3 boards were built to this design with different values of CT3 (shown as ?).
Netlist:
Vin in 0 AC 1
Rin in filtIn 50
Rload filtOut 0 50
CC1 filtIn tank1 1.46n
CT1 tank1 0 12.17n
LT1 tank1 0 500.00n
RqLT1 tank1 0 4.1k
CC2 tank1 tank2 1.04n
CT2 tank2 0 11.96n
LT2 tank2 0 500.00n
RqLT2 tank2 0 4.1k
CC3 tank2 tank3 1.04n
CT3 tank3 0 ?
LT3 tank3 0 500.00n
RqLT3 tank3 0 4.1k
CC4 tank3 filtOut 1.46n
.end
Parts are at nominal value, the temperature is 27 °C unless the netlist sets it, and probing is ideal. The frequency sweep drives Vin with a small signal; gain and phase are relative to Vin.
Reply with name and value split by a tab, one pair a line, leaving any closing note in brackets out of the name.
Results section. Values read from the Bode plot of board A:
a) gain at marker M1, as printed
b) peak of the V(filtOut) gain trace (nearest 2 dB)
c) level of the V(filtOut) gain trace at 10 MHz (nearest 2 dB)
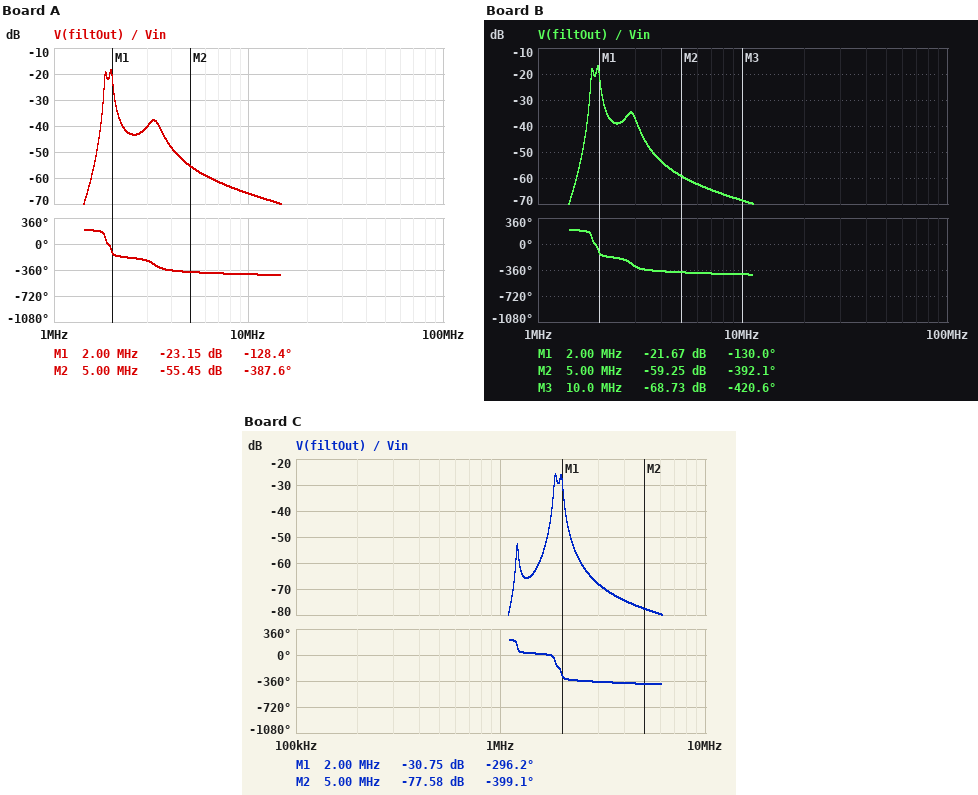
gain at marker M1, as printed	-23.15 dB
peak of the V(filtOut) gain trace	-18 dB
level of the V(filtOut) gain trace at 10 MHz	-66 dB
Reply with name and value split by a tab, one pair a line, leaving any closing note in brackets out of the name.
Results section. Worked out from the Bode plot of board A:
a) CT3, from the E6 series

CT3, from the E6 series	3.3 nF
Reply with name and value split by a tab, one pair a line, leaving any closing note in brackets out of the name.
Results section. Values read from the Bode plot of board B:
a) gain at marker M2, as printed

gain at marker M2, as printed	-59.25 dB
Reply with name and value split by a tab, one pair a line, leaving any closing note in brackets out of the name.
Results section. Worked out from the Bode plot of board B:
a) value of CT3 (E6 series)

value of CT3	4.7 nF
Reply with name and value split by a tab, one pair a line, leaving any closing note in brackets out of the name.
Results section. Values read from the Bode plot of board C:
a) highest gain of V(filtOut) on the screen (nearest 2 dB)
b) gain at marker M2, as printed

highest gain of V(filtOut) on the screen	-26 dB
gain at marker M2, as printed	-77.58 dB
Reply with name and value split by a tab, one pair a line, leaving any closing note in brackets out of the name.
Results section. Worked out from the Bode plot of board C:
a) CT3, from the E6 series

CT3, from the E6 series	33 nF
